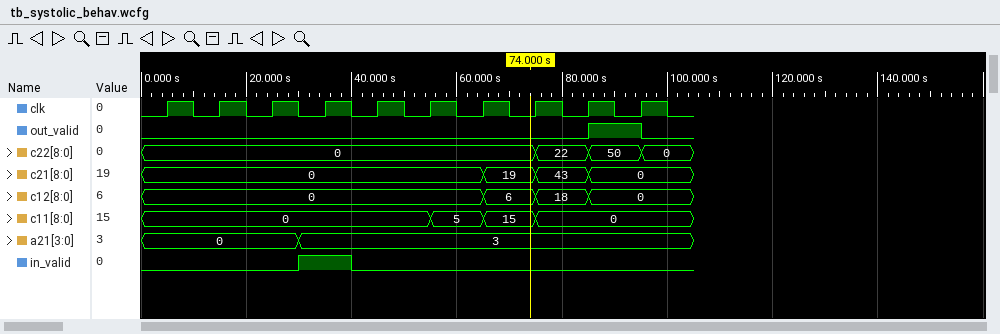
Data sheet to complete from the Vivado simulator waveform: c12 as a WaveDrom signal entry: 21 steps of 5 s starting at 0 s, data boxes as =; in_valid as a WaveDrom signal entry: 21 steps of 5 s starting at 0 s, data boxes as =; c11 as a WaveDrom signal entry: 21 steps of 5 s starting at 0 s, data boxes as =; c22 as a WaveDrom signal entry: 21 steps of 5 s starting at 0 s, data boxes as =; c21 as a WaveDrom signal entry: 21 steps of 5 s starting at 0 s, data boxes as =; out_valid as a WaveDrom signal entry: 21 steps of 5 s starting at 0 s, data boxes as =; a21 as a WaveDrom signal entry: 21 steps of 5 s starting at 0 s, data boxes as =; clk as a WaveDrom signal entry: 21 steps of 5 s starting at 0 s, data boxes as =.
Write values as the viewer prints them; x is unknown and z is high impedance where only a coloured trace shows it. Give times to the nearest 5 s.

{name: 'c12', wave: '=............=.=.=...', data: '0 6 18 0'}
{name: 'in_valid', wave: '0.....1.0............'}
{name: 'c11', wave: '=..........=.=.=.....', data: '0 5 15 0'}
{name: 'c22', wave: '=..............=.=.=.', data: '0 22 50 0'}
{name: 'c21', wave: '=............=.=.=...', data: '0 19 43 0'}
{name: 'out_valid', wave: '0................1.0.'}
{name: 'a21', wave: '=.....=..............', data: '0 3'}
{name: 'clk', wave: '010101010101010101010'}
